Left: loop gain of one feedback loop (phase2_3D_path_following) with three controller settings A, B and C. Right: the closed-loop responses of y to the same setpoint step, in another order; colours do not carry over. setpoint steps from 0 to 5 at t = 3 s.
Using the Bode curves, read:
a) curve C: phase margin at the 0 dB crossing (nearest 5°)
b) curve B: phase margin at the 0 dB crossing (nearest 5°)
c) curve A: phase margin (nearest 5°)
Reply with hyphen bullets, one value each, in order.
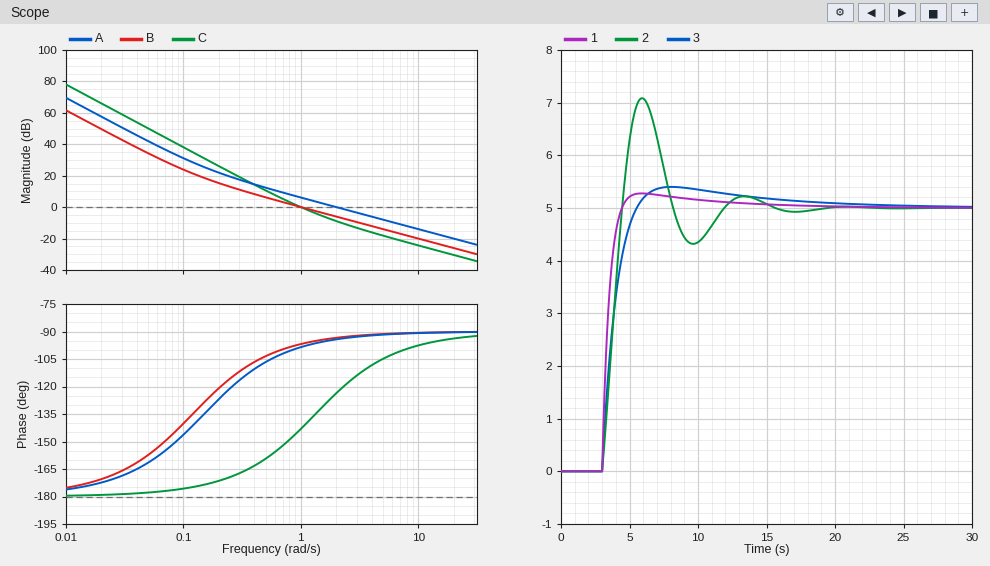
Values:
- 35°
- 85°
- 85°
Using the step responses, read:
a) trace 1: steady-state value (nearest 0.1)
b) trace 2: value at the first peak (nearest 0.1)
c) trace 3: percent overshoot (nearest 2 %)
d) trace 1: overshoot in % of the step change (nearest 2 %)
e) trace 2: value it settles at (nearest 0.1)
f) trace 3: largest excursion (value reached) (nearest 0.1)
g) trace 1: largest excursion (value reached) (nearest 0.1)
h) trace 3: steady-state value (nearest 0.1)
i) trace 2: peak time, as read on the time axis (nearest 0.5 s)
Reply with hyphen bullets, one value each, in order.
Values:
- 5.0
- 7.1
- 8 %
- 6 %
- 5.0
- 5.4
- 5.3
- 5.0
- 6.0 s
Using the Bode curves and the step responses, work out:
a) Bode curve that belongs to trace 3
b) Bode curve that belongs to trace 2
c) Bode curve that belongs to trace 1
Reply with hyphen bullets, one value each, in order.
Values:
- B
- C
- A
